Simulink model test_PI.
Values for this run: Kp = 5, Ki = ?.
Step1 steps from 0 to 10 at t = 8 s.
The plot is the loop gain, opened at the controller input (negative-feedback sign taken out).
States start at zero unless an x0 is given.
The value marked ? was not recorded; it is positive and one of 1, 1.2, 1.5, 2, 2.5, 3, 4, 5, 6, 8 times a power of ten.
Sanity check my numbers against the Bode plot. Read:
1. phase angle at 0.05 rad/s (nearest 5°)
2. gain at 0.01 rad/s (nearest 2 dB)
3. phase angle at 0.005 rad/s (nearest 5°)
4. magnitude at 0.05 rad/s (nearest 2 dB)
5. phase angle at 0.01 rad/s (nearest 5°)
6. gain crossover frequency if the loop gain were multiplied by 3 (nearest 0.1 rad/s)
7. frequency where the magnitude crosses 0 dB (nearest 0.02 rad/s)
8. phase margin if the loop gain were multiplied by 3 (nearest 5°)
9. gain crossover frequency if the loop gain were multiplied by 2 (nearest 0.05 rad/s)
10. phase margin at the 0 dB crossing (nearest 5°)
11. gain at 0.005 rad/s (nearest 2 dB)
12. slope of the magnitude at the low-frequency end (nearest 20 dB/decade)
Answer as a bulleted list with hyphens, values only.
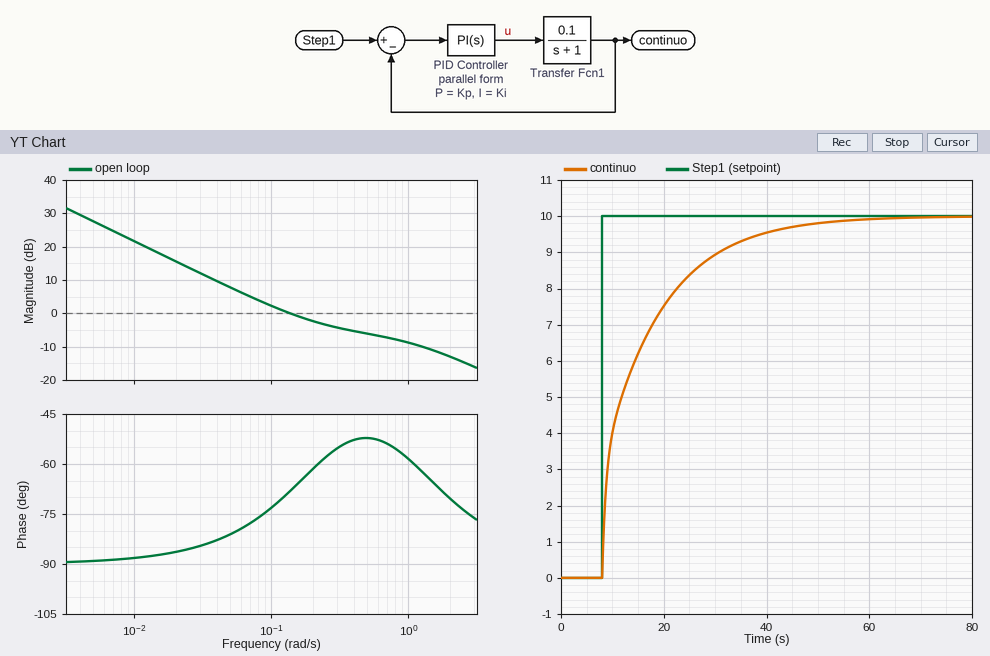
- -80°
- 22 dB
- -90°
- 8 dB
- -90°
- 1.2 rad/s
- 0.14 rad/s
- 120°
- 0.50 rad/s
- 110°
- 28 dB
- -20 dB/decade
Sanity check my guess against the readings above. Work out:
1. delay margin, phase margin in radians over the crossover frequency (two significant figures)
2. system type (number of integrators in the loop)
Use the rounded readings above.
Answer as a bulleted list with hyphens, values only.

- 14 s
- 1
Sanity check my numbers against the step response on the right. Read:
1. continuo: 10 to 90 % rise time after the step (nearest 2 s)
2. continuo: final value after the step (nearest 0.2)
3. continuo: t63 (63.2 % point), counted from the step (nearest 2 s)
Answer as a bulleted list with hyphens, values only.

- 22 s
- 10.0
- 8 s
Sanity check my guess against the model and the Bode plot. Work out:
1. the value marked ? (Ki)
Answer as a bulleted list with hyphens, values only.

- 1.2
